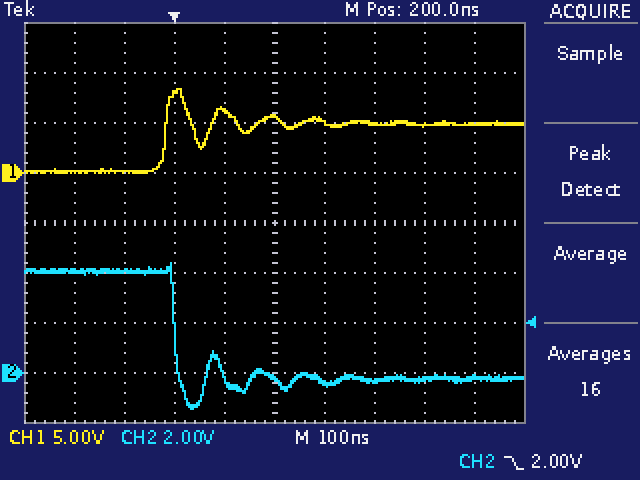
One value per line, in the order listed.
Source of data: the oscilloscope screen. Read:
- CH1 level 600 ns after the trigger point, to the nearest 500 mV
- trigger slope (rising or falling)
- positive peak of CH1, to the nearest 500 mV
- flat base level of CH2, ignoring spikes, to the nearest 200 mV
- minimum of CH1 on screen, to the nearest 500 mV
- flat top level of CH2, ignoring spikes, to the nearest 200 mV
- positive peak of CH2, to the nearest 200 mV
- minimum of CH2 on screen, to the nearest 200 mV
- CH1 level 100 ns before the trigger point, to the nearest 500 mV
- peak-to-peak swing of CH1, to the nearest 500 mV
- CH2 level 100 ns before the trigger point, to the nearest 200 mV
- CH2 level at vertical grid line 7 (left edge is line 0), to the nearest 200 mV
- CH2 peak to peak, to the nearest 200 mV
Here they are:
5.0 V
falling
8.5 V
-200 mV
0.0 V
4.0 V
4.4 V
-1.4 V
0.0 V
8.5 V
4.0 V
-400 mV
5.8 V
